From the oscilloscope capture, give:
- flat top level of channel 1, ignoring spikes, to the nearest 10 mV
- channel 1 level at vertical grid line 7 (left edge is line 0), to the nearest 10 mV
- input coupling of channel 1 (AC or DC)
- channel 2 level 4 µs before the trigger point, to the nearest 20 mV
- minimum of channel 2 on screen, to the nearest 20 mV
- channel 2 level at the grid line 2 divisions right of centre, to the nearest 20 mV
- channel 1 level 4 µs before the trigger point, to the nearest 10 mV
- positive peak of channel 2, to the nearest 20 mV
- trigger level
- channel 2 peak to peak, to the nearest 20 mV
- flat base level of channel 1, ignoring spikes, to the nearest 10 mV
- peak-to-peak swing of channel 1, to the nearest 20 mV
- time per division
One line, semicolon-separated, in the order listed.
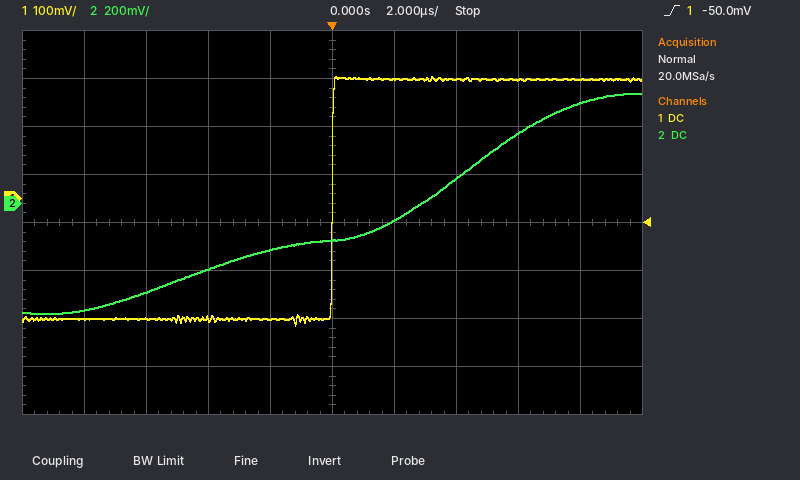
250 mV; 250 mV; DC; -280 mV; -460 mV; 100 mV; -250 mV; 460 mV; -50.0 mV; 920 mV; -250 mV; 520 mV; 2 µs
